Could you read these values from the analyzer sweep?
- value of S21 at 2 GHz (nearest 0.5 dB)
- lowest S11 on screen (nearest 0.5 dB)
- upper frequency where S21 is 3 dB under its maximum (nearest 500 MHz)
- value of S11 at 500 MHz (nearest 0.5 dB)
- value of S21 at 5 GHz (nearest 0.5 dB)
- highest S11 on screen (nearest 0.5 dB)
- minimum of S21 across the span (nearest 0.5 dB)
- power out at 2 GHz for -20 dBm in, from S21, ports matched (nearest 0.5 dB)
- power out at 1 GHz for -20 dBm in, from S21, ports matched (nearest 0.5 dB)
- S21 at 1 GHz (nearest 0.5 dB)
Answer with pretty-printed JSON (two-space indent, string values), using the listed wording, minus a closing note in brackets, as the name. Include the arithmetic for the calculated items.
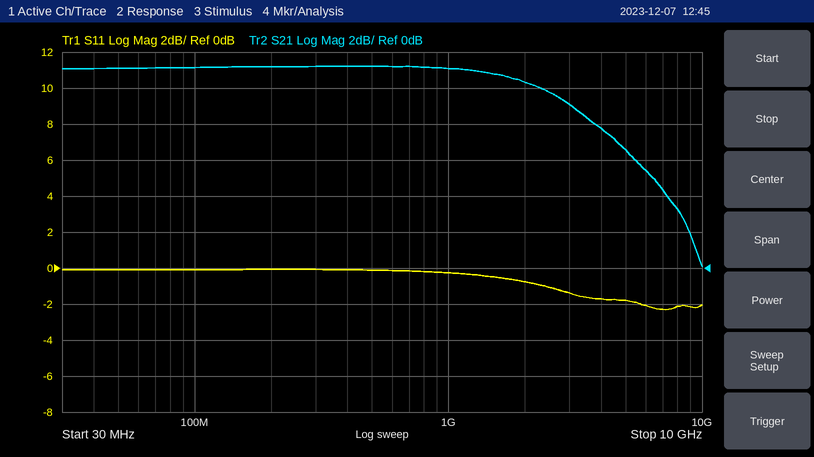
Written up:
{
  "value of S21 at 2 GHz": "10.5 dB",
  "lowest S11 on screen": "-2.5 dB",
  "upper frequency where S21 is 3 dB under its maximum": "3.5 GHz",
  "value of S11 at 500 MHz": "0.0 dB",
  "value of S21 at 5 GHz": "6.5 dB",
  "highest S11 on screen": "0.0 dB",
  "minimum of S21 across the span": "0.0 dB",
  "power out at 2 GHz for -20 dBm in, from S21, ports matched": "-20 dBm + (10.5 dB) = -9.5 dBm",
  "power out at 1 GHz for -20 dBm in, from S21, ports matched": "-20 dBm + (11.0 dB) = -9.0 dBm",
  "S21 at 1 GHz": "11.0 dB"
}
